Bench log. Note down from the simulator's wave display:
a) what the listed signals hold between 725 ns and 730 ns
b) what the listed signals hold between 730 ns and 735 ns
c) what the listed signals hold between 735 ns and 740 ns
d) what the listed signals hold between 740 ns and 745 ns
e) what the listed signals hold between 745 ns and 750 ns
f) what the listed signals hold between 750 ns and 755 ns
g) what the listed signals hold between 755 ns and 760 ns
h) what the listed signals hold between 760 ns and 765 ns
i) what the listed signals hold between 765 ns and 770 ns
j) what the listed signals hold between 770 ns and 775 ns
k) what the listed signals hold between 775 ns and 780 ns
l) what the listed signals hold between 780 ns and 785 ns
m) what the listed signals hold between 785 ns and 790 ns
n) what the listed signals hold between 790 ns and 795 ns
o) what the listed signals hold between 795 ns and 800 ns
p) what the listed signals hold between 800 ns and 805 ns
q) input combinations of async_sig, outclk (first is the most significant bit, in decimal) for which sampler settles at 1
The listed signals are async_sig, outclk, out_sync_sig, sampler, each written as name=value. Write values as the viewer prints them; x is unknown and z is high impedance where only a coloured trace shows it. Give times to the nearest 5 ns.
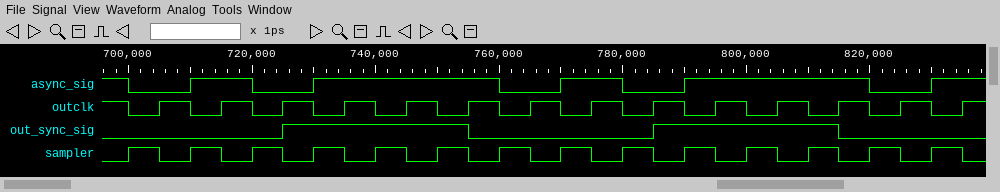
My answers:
async_sig=0, outclk=1, out_sync_sig=1, sampler=0
async_sig=1, outclk=0, out_sync_sig=1, sampler=1
async_sig=1, outclk=1, out_sync_sig=1, sampler=0
async_sig=1, outclk=0, out_sync_sig=1, sampler=1
async_sig=1, outclk=1, out_sync_sig=1, sampler=0
async_sig=1, outclk=0, out_sync_sig=1, sampler=1
async_sig=1, outclk=1, out_sync_sig=0, sampler=0
async_sig=0, outclk=0, out_sync_sig=0, sampler=1
async_sig=0, outclk=1, out_sync_sig=0, sampler=0
async_sig=1, outclk=0, out_sync_sig=0, sampler=1
async_sig=1, outclk=1, out_sync_sig=0, sampler=0
async_sig=0, outclk=0, out_sync_sig=0, sampler=1
async_sig=0, outclk=1, out_sync_sig=1, sampler=0
async_sig=1, outclk=0, out_sync_sig=1, sampler=1
async_sig=1, outclk=1, out_sync_sig=1, sampler=0
async_sig=1, outclk=0, out_sync_sig=1, sampler=1
0, 2
